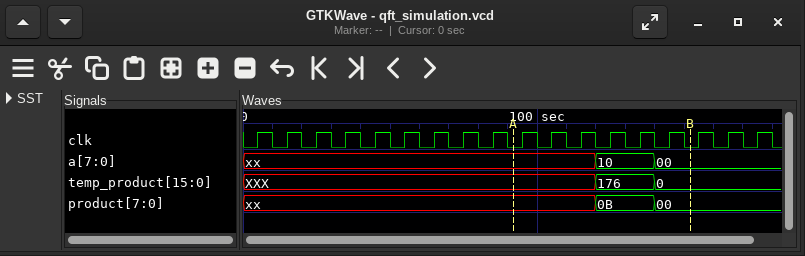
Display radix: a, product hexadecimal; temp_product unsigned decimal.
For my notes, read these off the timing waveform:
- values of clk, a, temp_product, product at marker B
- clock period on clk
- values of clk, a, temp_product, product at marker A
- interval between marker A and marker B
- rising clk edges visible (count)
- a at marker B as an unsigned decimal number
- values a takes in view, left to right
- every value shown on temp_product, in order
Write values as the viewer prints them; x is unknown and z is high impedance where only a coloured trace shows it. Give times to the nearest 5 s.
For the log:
clk=0, a=00, temp_product=0, product=00
10 s
clk=0, a=xx, temp_product=XXX, product=xx
60 s
18
0
xx, 10, 00
XXX, 176, 0
